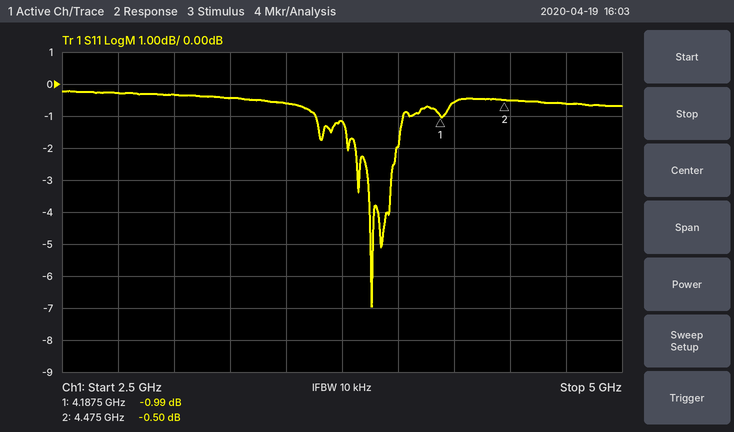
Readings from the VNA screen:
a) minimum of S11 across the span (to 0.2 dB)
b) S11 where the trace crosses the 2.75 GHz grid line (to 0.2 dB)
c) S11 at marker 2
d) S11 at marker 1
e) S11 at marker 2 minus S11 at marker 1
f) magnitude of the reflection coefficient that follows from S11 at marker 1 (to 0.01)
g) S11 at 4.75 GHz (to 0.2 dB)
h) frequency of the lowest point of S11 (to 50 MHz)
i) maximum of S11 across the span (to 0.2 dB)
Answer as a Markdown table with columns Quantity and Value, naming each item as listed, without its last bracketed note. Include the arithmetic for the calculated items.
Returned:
| Quantity | Value |
|---|---|
| minimum of S11 across the span | -7.0 dB |
| S11 where the trace crosses the 2.75 GHz grid line | -0.2 dB |
| S11 at marker 2 | -0.50 dB |
| S11 at marker 1 | -0.99 dB |
| S11 at marker 2 minus S11 at marker 1 | -0.5 − (-0.99) = 0.49 dB |
| magnitude of the reflection coefficient that follows from S11 at marker 1 | 10^(-0.99/20) ≈ 0.89 |
| S11 at 4.75 GHz | -0.6 dB |
| frequency of the lowest point of S11 | 3.90 GHz |
| maximum of S11 across the span | -0.2 dB |
